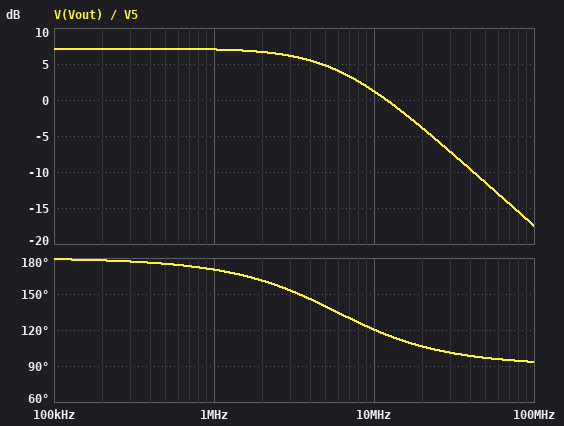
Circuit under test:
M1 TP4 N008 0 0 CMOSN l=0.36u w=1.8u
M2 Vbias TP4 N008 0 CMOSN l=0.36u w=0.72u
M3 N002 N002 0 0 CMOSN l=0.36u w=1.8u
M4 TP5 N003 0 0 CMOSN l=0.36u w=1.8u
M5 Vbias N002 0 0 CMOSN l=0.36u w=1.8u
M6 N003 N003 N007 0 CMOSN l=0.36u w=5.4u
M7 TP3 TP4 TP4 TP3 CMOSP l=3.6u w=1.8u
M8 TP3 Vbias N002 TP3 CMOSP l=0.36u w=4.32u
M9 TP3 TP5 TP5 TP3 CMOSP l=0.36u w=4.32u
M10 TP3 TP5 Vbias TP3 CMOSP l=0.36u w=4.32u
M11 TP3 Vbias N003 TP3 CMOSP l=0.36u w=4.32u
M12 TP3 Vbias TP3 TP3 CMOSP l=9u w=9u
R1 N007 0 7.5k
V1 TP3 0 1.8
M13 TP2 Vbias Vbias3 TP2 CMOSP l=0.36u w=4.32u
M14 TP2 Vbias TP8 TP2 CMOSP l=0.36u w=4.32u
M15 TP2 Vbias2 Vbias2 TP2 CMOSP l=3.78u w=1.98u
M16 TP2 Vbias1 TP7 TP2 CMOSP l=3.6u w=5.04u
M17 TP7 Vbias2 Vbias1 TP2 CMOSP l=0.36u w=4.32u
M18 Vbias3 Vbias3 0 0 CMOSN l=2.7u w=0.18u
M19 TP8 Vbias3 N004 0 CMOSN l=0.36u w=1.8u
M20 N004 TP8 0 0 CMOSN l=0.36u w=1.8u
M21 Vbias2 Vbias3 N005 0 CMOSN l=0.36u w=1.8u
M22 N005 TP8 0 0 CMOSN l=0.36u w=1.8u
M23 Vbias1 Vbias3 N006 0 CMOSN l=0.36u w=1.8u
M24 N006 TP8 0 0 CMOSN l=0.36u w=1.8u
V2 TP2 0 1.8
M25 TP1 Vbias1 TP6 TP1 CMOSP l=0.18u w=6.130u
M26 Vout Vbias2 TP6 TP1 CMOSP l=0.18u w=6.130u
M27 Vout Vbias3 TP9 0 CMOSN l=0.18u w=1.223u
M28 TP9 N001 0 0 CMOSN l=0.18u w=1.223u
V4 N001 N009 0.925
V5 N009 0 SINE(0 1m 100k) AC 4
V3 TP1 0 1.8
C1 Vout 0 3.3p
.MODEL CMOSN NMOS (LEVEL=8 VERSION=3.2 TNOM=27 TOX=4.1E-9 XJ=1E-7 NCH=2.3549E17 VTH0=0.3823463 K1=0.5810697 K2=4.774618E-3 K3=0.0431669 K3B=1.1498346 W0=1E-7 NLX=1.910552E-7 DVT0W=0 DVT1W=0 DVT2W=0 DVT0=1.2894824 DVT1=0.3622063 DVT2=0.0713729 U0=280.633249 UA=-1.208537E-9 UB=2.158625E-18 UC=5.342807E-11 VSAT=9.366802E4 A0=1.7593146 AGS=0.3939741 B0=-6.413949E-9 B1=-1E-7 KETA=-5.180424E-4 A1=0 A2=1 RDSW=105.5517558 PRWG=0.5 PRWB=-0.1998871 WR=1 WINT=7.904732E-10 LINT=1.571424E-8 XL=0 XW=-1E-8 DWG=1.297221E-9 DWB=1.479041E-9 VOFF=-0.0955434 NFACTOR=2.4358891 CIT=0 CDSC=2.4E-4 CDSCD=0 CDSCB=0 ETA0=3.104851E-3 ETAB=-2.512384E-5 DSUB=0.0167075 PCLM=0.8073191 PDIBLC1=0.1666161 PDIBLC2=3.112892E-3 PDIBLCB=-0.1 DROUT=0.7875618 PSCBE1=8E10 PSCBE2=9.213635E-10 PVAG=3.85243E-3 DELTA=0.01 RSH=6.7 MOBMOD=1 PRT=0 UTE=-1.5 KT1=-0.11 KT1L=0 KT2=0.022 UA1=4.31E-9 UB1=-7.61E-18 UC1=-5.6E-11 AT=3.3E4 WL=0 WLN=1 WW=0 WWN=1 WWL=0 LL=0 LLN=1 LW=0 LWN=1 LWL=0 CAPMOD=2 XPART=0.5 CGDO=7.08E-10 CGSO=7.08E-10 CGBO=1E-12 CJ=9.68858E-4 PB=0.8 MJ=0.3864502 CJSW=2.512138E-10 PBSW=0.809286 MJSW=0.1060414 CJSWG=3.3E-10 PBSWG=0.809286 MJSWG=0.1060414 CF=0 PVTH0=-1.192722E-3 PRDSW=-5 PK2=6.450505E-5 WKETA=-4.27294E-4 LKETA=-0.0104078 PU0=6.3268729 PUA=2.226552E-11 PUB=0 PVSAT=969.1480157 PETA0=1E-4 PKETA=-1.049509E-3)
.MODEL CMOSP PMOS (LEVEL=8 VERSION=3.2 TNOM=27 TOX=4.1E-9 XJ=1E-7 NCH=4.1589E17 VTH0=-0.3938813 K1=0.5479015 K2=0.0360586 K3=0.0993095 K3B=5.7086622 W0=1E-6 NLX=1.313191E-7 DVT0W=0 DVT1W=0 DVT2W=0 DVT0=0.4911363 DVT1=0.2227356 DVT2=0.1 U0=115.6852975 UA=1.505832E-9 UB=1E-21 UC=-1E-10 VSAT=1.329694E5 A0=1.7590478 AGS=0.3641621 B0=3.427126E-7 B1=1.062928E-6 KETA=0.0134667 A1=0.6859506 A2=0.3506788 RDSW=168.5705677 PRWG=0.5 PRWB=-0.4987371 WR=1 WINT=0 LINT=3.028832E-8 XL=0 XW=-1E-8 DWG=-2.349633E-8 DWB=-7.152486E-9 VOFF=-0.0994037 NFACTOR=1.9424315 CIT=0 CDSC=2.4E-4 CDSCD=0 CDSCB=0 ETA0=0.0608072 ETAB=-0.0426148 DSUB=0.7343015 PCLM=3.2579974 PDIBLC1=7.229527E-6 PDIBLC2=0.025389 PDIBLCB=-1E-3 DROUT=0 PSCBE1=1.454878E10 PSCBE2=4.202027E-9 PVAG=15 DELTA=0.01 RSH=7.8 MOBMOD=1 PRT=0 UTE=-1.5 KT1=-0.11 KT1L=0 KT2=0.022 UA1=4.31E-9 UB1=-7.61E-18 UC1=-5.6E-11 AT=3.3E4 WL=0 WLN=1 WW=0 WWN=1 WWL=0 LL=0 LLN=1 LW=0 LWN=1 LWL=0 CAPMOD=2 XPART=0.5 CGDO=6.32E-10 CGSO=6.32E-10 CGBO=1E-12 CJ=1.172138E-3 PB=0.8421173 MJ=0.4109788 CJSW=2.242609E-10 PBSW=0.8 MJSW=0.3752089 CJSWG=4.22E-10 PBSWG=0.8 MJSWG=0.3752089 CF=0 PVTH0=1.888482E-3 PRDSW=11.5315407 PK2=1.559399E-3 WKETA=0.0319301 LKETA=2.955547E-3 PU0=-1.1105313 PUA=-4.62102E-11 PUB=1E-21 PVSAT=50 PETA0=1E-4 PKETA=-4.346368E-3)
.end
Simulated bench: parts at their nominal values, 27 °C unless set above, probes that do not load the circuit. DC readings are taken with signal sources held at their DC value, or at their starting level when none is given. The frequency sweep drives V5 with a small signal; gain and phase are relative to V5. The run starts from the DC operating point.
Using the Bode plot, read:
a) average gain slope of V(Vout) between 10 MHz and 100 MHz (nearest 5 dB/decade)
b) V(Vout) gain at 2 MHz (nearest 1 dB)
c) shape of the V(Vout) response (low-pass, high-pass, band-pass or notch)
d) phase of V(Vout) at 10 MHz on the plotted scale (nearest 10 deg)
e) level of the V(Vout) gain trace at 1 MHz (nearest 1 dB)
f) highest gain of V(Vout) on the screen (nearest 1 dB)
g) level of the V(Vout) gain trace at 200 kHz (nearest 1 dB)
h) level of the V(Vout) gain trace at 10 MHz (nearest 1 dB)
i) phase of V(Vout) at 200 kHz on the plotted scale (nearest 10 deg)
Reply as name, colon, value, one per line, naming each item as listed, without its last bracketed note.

average gain slope of V(Vout) between 10 MHz and 100 MHz: -20 dB/decade
V(Vout) gain at 2 MHz: 7 dB
shape of the V(Vout) response: low-pass
phase of V(Vout) at 10 MHz on the plotted scale: 120 deg
level of the V(Vout) gain trace at 1 MHz: 7 dB
highest gain of V(Vout) on the screen: 7 dB
level of the V(Vout) gain trace at 200 kHz: 7 dB
level of the V(Vout) gain trace at 10 MHz: 1 dB
phase of V(Vout) at 200 kHz on the plotted scale: 180 deg
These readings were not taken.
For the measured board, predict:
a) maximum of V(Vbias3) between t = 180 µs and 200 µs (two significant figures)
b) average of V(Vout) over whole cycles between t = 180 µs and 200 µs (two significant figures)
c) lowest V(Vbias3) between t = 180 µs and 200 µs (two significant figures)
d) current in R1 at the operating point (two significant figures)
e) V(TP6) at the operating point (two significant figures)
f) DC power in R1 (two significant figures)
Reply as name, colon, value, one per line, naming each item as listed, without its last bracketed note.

maximum of V(Vbias3) between t = 180 µs and 200 µs: 1.3 V
average of V(Vout) over whole cycles between t = 180 µs and 200 µs: 360 mV
lowest V(Vbias3) between t = 180 µs and 200 µs: 1.3 V
current in R1 at the operating point: 6.2 µA
V(TP6) at the operating point: 1.5 V
DC power in R1: 290 nW
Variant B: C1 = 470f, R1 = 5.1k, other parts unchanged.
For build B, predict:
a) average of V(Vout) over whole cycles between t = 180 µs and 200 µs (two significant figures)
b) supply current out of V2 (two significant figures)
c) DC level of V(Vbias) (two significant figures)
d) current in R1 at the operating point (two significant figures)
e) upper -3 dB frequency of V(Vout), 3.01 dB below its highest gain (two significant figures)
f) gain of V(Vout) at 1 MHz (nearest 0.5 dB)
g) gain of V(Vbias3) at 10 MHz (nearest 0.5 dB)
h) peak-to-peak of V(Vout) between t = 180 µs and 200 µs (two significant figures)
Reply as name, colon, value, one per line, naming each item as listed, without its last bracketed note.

average of V(Vout) over whole cycles between t = 180 µs and 200 µs: 1.6 V
supply current out of V2: 39 µA
DC level of V(Vbias): 1.2 V
current in R1 at the operating point: 10 µA
upper -3 dB frequency of V(Vout), 3.01 dB below its highest gain: 120 MHz
gain of V(Vout) at 1 MHz: 1.5 dB
gain of V(Vbias3) at 10 MHz: -40.0 dB
peak-to-peak of V(Vout) between t = 180 µs and 200 µs: 2.4 mV
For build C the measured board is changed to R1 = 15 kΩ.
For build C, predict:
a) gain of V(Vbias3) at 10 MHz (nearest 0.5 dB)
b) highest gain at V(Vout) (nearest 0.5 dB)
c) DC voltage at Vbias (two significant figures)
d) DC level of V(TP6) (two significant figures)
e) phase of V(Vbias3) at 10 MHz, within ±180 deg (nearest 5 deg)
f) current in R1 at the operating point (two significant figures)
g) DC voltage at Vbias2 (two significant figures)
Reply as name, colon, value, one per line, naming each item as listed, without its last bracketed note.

gain of V(Vbias3) at 10 MHz: -53.5 dB
highest gain at V(Vout): -19.0 dB
DC voltage at Vbias: 1.3 V
DC level of V(TP6): 1.6 V
phase of V(Vbias3) at 10 MHz, within ±180 deg: -120 deg
current in R1 at the operating point: 2.7 µA
DC voltage at Vbias2: 950 mV
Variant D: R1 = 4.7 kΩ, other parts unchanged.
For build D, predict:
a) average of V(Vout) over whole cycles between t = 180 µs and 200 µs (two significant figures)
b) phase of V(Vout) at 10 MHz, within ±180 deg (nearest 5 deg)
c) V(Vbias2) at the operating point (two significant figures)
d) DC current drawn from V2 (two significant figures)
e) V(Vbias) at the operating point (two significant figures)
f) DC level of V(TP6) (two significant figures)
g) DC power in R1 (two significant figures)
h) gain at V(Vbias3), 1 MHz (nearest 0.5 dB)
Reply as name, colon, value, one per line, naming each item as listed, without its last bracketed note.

average of V(Vout) over whole cycles between t = 180 µs and 200 µs: 1.6 V
phase of V(Vout) at 10 MHz, within ±180 deg: 155 deg
V(Vbias2) at the operating point: 450 mV
DC current drawn from V2: 44 µA
V(Vbias) at the operating point: 1.2 V
DC level of V(TP6): 1.7 V
DC power in R1: 620 nW
gain at V(Vbias3), 1 MHz: -62.0 dB
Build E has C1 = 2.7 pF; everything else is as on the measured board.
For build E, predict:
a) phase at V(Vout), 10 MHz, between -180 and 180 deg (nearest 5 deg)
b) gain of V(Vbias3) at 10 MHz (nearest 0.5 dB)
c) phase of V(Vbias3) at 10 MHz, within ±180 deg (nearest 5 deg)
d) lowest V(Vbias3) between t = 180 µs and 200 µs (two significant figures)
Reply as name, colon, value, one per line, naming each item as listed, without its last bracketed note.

phase at V(Vout), 10 MHz, between -180 and 180 deg: 125 deg
gain of V(Vbias3) at 10 MHz: -35.5 dB
phase of V(Vbias3) at 10 MHz, within ±180 deg: -140 deg
lowest V(Vbias3) between t = 180 µs and 200 µs: 1.3 V
